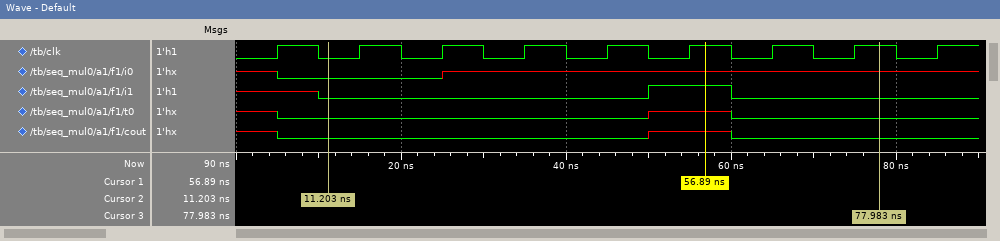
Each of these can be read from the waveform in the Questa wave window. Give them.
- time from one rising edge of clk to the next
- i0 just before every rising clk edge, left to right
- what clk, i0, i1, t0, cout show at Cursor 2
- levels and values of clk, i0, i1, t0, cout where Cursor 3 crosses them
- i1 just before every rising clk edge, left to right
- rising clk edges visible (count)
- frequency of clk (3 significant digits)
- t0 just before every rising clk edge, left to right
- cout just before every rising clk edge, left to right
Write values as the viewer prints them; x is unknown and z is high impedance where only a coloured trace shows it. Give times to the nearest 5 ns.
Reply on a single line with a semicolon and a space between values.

10 ns; x 0 0 x x x x x x; clk=0, i0=0, i1=0, t0=0, cout=0; clk=1, i0=x, i1=0, t0=0, cout=0; x 0 0 0 0 1 0 0 0; 9; 100 MHz; x 0 0 0 0 x 0 0 0; x 0 0 0 0 x 0 0 0
